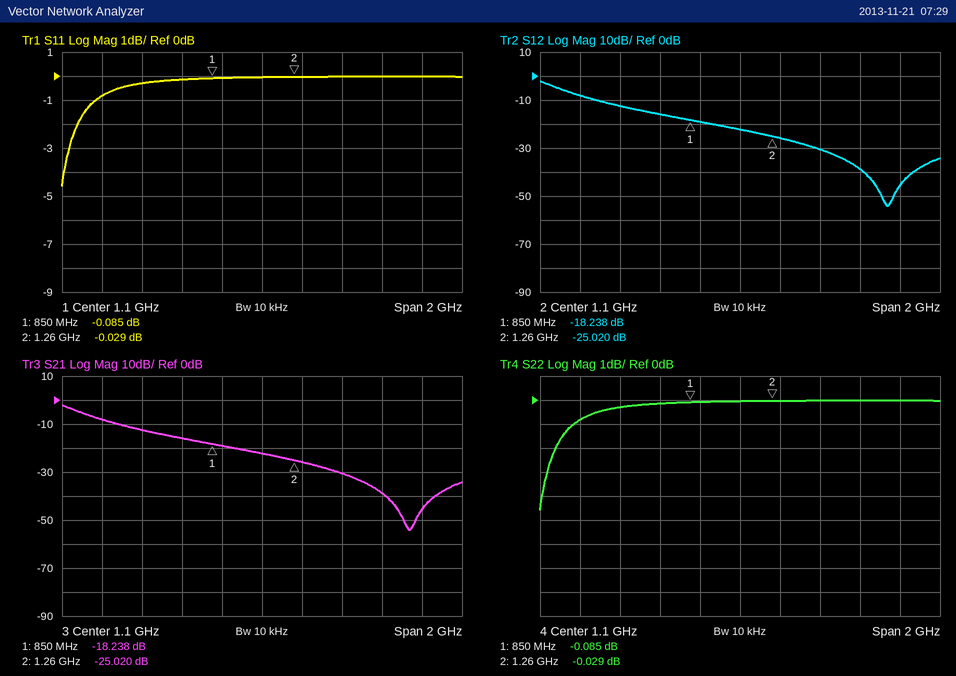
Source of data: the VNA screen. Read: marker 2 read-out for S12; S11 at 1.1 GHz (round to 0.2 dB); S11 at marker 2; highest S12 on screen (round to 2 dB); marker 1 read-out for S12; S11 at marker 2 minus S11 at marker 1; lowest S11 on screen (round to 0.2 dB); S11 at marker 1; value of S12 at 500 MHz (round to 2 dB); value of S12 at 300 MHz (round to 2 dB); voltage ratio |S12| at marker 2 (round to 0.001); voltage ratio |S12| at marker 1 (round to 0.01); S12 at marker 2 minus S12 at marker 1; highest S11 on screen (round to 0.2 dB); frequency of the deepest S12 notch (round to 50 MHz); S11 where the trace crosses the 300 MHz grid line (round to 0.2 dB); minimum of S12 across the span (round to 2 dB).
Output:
-25.020 dB
0.0 dB
-0.029 dB
-2 dB
-18.238 dB
0.056 dB
-4.6 dB
-0.085 dB
-12 dB
-8 dB
0.056
0.12
-6.782 dB
0.0 dB
1.85 GHz
-0.8 dB
-54 dB
